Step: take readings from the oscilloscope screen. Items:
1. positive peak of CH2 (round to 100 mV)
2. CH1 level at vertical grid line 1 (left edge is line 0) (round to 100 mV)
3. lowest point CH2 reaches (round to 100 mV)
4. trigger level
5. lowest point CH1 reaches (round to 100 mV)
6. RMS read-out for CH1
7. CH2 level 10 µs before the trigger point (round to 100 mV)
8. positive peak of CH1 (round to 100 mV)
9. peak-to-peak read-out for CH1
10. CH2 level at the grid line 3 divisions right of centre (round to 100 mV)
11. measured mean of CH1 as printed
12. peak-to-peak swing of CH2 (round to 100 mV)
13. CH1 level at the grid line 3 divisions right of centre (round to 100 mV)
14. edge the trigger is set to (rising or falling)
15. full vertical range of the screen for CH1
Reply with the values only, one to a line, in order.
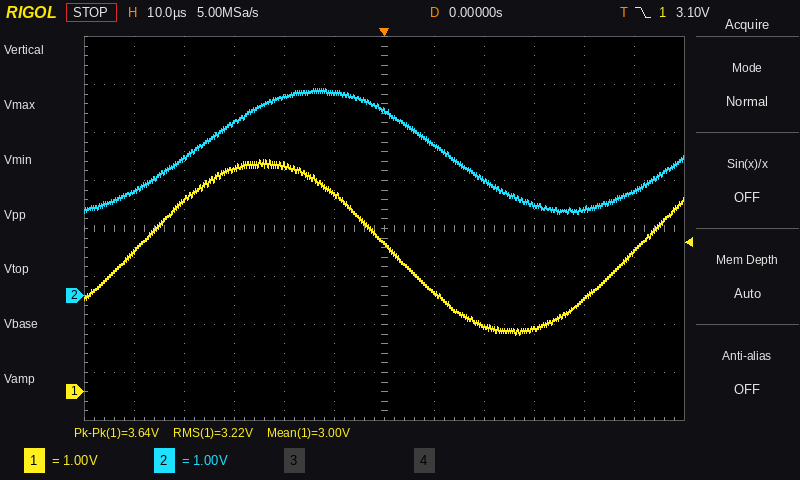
4.3 V
2.9 V
1.7 V
3.10 V
1.2 V
3.22 V
4.2 V
4.8 V
3.64 V
1.9 V
3.00 V
2.6 V
1.3 V
falling
8 V
